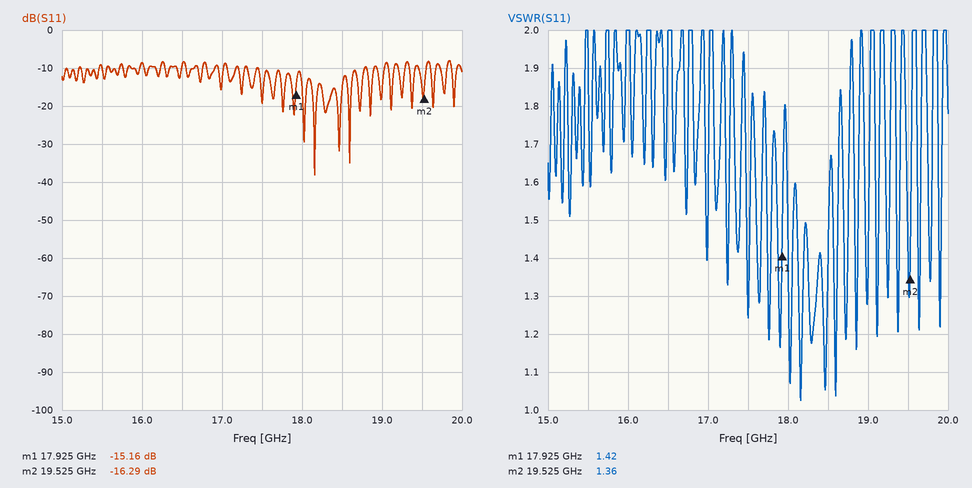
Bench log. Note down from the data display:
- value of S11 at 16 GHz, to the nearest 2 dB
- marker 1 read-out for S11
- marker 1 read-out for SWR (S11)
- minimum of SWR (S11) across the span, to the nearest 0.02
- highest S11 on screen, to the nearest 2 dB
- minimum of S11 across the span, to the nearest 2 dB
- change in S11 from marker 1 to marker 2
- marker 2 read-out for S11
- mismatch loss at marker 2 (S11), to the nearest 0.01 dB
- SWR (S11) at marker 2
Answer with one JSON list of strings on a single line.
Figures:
["-8 dB", "-15.16 dB", "1.42", "1.02", "-8 dB", "-38 dB", "-1.13 dB", "-16.29 dB", "0.10 dB", "1.36"]
